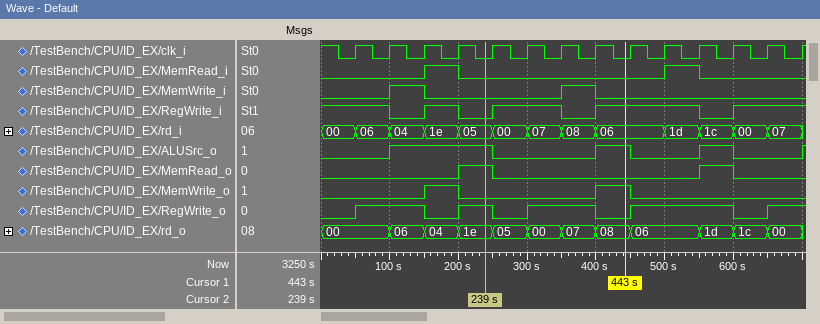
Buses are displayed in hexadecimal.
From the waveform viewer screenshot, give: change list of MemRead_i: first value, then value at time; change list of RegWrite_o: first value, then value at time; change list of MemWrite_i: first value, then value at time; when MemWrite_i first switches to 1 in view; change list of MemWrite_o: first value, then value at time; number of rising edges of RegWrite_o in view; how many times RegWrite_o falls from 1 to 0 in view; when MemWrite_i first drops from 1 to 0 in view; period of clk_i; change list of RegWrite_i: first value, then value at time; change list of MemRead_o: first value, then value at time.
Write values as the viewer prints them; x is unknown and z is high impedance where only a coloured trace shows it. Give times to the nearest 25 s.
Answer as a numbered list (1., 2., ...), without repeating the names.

1. 0, 1 at 150 s, 0 at 200 s, 1 at 500 s, 0 at 550 s
2. 0, 1 at 50 s, 0 at 150 s, 1 at 200 s, 0 at 250 s, 1 at 300 s, 0 at 400 s, 1 at 450 s, 0 at 600 s, 1 at 650 s
3. 0, 1 at 100 s, 0 at 150 s, 1 at 350 s, 0 at 400 s
4. 100 s
5. 0, 1 at 150 s, 0 at 200 s, 1 at 400 s, 0 at 450 s
6. 5
7. 4
8. 150 s
9. 50 s
10. 1, 0 at 100 s, 1 at 150 s, 0 at 200 s, 1 at 250 s, 0 at 350 s, 1 at 400 s, 0 at 550 s, 1 at 600 s
11. 0, 1 at 200 s, 0 at 250 s, 1 at 550 s, 0 at 600 s
